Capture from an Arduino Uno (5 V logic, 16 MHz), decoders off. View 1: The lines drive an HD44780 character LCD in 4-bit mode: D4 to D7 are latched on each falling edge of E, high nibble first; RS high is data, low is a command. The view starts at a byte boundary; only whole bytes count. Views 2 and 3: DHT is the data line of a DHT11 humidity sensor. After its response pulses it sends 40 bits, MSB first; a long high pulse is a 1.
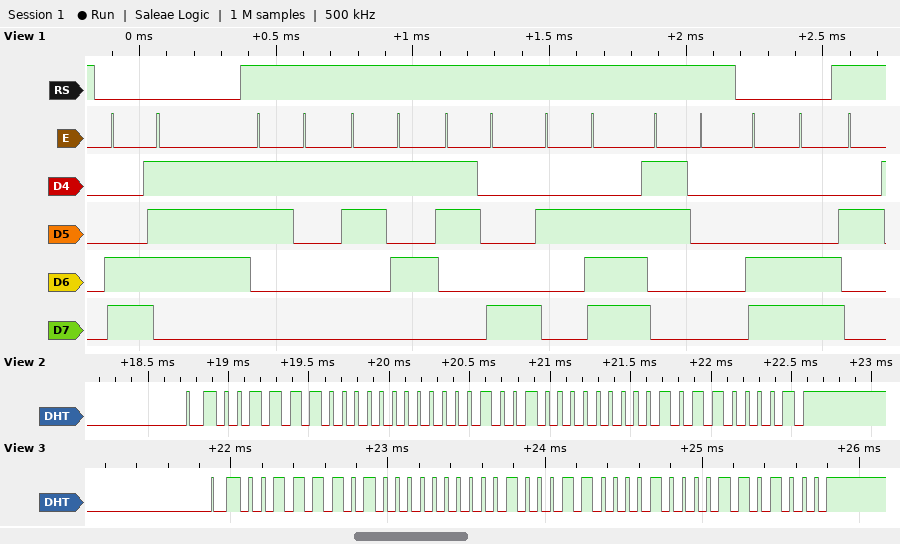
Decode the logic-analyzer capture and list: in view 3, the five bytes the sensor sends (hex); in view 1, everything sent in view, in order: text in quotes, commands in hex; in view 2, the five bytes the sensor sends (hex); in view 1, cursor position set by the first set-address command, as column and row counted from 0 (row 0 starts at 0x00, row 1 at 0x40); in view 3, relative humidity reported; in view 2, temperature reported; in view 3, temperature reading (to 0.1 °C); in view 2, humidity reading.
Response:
3D 00 23 08 68
0xC7 "158.0" 0xCC
3C 00 24 01 61
column 7, row 1
61 %
36.1 °C
35.8 °C
60 %
